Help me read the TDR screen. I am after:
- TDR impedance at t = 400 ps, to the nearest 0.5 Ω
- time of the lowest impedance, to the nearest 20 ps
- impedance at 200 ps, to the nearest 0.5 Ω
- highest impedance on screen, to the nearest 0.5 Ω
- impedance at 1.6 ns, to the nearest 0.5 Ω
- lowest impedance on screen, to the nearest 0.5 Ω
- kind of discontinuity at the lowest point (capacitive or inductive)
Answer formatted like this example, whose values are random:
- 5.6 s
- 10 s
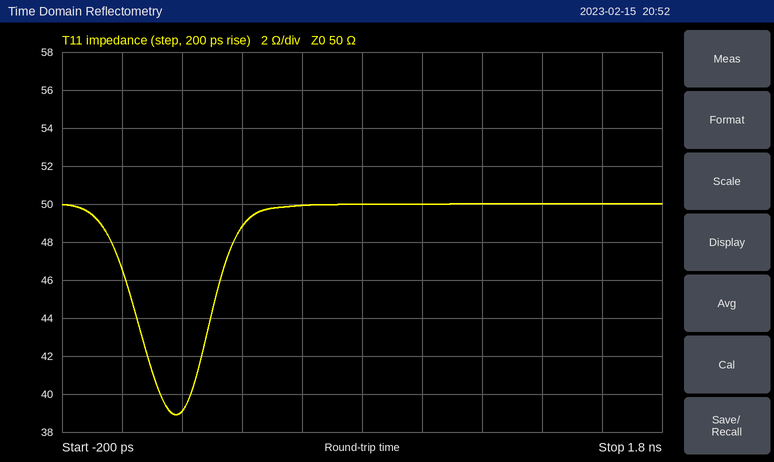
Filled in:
- 49.0 Ω
- 180 ps
- 39.0 Ω
- 50.0 Ω
- 50.0 Ω
- 39.0 Ω
- capacitive
